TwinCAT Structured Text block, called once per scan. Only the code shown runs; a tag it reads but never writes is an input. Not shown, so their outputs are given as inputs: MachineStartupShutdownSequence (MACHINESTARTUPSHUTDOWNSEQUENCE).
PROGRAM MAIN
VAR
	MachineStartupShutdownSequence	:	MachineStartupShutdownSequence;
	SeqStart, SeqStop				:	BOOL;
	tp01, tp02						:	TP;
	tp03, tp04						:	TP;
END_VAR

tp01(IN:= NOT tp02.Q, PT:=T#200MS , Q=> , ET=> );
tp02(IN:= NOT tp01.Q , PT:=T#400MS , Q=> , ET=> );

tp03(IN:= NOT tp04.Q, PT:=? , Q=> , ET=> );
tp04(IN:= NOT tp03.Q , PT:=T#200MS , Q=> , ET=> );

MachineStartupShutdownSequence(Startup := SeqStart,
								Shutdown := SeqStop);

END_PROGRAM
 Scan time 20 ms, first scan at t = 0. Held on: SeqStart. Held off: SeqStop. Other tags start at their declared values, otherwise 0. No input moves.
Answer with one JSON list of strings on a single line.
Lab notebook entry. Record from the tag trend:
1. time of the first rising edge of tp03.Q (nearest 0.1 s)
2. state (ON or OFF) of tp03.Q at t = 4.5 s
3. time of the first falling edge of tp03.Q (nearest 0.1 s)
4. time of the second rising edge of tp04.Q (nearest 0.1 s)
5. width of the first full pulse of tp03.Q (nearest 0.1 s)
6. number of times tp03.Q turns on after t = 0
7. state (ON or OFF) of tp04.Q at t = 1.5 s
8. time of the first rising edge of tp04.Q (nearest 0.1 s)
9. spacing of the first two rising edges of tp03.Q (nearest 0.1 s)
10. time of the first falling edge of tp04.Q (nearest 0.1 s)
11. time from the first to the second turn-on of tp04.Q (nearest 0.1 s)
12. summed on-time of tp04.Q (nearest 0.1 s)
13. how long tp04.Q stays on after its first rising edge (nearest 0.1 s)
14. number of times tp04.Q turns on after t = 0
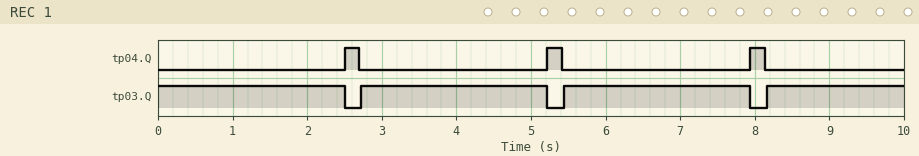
["2.7 s", "ON", "2.5 s", "5.2 s", "2.5 s", "3", "OFF", "2.5 s", "2.7 s", "2.7 s", "2.7 s", "0.6 s", "0.2 s", "3"]
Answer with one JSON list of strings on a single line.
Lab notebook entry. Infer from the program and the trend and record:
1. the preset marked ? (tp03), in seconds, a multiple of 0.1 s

["2.5 s"]
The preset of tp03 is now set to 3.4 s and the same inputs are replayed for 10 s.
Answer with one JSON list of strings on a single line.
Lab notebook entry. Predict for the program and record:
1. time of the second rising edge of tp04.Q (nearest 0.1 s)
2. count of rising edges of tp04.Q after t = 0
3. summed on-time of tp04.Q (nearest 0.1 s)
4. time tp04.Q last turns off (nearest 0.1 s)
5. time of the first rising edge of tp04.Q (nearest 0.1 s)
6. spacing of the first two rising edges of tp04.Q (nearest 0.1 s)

["7.0 s", "2", "0.4 s", "7.2 s", "3.4 s", "3.6 s"]
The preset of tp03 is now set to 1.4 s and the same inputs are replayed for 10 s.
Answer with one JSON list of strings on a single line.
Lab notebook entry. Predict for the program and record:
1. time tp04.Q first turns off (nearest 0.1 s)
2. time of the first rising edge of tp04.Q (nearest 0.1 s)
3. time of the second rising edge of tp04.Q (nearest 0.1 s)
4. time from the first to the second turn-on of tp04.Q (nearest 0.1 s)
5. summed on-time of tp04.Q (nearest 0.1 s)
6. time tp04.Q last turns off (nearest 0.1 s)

["1.6 s", "1.4 s", "3.0 s", "1.6 s", "1.2 s", "9.7 s"]
